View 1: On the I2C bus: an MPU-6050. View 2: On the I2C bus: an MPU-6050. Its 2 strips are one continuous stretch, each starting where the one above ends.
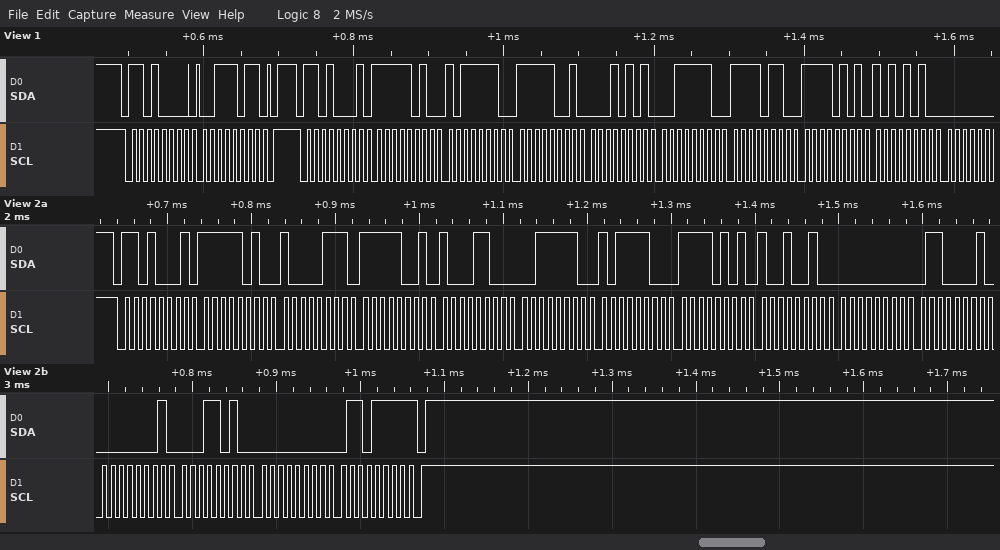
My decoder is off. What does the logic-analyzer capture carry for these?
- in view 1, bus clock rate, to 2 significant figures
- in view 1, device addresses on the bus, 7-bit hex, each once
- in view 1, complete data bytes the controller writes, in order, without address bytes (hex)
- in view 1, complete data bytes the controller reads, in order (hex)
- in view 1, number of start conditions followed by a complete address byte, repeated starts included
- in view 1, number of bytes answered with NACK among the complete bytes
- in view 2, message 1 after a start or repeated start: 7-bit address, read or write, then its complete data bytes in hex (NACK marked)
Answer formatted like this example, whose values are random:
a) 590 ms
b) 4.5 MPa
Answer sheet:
a) 100 kHz
b) 0x68
c) 3B
d) FA BE F9 15 3E F6 F5 AA
e) 2
f) 0
g) 0x68 read: FA 87 F9 8C 3E BC F5 92 00 61 01 1A 00 6F NACK
